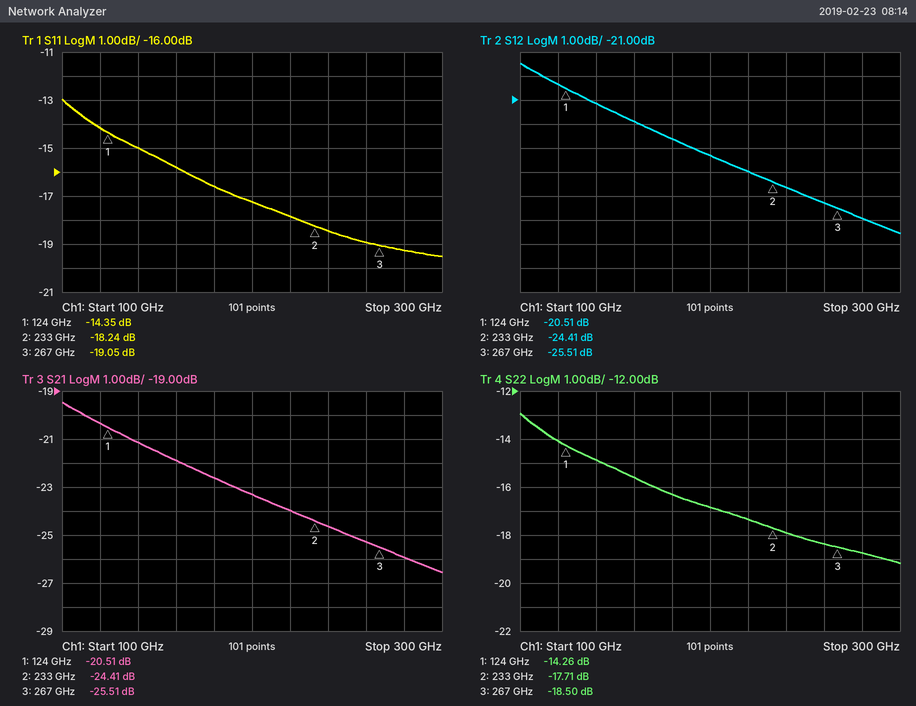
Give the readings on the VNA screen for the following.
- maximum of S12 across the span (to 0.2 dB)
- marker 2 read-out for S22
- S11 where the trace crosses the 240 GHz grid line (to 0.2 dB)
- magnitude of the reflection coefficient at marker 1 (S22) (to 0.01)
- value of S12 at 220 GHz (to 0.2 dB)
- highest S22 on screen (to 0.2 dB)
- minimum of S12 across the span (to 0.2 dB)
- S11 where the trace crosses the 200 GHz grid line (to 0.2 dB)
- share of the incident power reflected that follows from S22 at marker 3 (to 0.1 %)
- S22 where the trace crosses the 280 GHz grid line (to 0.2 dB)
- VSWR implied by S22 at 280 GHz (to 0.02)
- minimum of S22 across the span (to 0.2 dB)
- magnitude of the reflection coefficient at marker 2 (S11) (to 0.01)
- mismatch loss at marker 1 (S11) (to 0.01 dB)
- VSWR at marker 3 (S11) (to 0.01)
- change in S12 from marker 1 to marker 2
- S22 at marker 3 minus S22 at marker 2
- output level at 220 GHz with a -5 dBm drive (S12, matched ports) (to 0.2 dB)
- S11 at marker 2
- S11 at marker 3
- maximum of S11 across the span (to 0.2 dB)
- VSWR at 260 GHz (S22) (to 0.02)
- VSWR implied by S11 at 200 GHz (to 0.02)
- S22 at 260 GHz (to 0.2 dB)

-19.4 dB
-17.71 dB
-18.4 dB
0.19
-24.0 dB
-13.0 dB
-26.6 dB
-17.2 dB
1.4 %
-18.8 dB
1.26
-19.2 dB
0.12
0.16 dB
1.25
-3.90 dB
-0.79 dB
-29.0 dBm
-18.24 dB
-19.05 dB
-13.0 dB
1.28
1.32
-18.4 dB
